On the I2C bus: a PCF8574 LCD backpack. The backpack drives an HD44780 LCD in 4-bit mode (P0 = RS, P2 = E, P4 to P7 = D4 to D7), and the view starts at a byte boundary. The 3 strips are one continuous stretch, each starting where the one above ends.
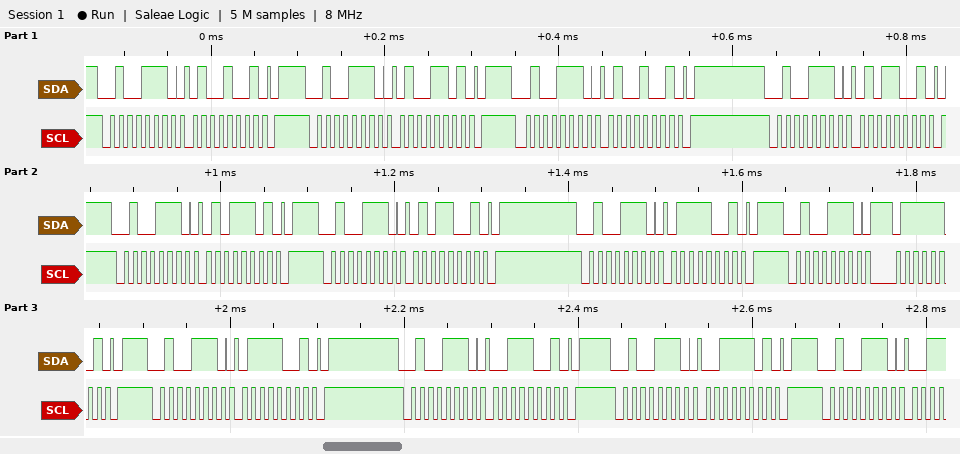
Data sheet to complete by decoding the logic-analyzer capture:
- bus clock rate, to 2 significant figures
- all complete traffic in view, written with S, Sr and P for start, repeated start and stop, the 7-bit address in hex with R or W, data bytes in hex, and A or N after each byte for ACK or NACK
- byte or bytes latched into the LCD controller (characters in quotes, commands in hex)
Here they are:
100 kHz
S 27W A 49 A P S 27W A 4D A P S 27W A 49 A P S 27W A 59 A P S 27W A 5D A P S 27W A 59 A P S 27W A 79 A P S 27W A 7D A P S 27W A 79 A P S 27W A 39 A P S 27W A 3D A P S 27W A
'E'
